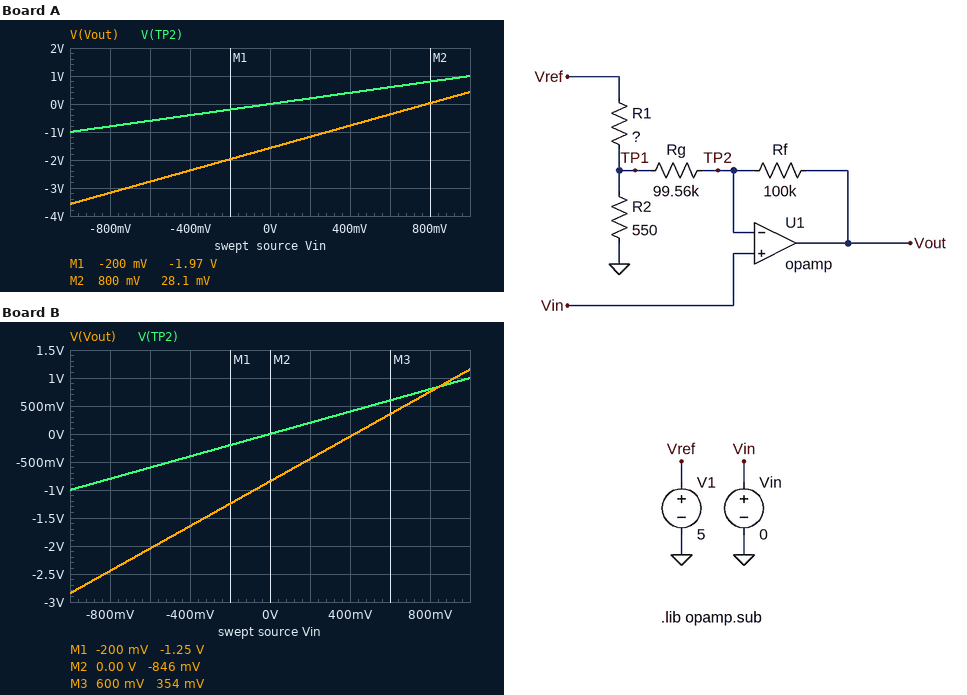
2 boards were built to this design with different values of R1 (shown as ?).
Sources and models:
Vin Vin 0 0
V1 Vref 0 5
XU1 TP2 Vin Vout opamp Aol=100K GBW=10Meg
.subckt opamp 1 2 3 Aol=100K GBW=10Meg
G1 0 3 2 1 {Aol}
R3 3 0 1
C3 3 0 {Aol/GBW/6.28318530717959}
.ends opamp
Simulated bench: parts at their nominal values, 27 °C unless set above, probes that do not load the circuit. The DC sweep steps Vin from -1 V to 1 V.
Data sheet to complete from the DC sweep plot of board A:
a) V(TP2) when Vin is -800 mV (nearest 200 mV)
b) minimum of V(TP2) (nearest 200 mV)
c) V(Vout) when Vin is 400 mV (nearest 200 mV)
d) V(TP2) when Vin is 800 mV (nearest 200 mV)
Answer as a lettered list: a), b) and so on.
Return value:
a) -800 mV
b) -1.0 V
c) -800 mV
d) 800 mV
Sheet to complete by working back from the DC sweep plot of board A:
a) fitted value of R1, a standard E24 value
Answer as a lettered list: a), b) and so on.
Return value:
a) 1.2 kΩ
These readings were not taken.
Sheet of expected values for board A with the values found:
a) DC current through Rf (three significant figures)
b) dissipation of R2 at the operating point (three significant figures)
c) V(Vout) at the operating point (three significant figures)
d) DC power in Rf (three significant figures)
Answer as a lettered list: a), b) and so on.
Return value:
a) 15.7 µA
b) 4.46 mW
c) -1.57 V
d) 24.7 µW
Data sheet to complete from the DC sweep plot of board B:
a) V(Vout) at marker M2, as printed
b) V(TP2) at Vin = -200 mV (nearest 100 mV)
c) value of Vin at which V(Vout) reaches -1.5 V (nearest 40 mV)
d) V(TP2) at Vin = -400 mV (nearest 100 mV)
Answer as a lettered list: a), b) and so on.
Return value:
a) -846 mV
b) -200 mV
c) -320 mV
d) -400 mV
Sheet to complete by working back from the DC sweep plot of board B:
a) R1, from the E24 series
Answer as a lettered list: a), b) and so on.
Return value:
a) 2.7 kΩ
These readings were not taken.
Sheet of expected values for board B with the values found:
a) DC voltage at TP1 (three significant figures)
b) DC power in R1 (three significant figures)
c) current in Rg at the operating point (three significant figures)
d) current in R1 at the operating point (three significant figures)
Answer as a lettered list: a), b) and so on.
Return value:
a) 842 mV
b) 6.40 mW
c) 8.46 µA
d) 1.54 mA
